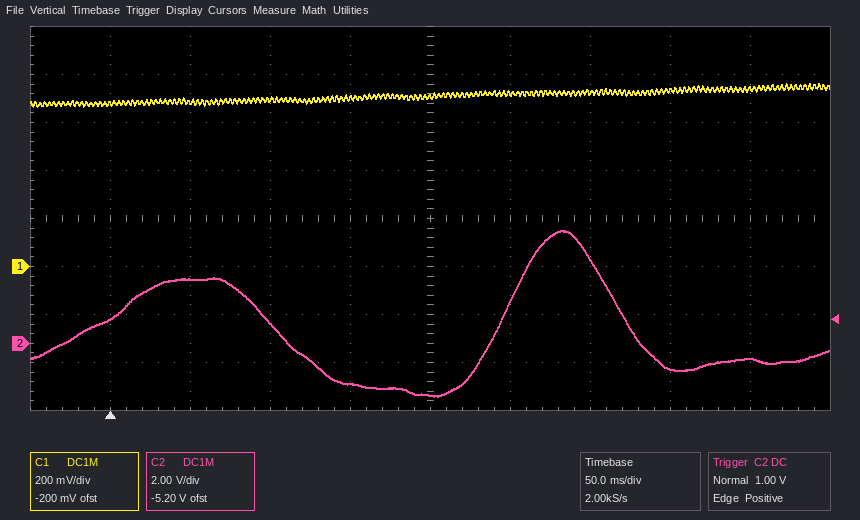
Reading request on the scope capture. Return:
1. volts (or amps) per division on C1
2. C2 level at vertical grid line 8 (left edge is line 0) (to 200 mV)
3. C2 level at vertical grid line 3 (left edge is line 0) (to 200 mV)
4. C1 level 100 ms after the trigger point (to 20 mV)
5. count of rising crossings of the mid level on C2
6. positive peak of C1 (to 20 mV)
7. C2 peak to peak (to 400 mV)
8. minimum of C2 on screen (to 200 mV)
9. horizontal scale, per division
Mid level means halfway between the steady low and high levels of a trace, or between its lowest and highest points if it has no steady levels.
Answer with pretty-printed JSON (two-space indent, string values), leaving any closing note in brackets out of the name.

{
  "volts (or amps) per division on C1": "200 mV",
  "C2 level at vertical grid line 8 (left edge is line 0)": "-1.0 V",
  "C2 level at vertical grid line 3 (left edge is line 0)": "800 mV",
  "C1 level 100 ms after the trigger point": "700 mV",
  "count of rising crossings of the mid level on C2": "2",
  "positive peak of C1": "760 mV",
  "C2 peak to peak": "6.8 V",
  "minimum of C2 on screen": "-2.2 V",
  "horizontal scale, per division": "50 ms"
}
